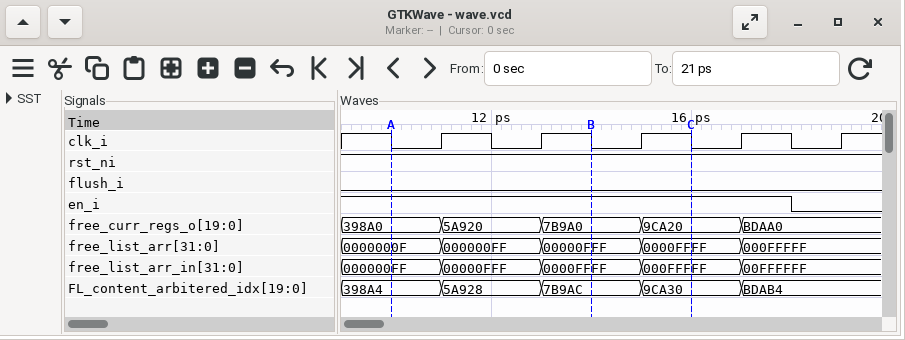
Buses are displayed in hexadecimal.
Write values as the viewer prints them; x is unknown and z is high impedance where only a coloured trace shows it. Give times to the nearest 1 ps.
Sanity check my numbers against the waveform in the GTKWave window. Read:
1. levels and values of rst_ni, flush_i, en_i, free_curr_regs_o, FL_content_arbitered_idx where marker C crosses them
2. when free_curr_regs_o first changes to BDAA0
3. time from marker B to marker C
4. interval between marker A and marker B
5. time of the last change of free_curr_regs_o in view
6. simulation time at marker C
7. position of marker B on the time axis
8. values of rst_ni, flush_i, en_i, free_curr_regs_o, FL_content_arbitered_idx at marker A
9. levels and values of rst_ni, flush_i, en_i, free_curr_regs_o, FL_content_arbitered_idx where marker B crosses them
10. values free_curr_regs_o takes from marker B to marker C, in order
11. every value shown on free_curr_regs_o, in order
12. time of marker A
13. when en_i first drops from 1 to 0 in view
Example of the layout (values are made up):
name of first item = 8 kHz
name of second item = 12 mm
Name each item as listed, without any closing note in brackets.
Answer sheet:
levels and values of rst_ni, flush_i, en_i, free_curr_regs_o, FL_content_arbitered_idx where marker C crosses them = rst_ni=1, flush_i=0, en_i=1, free_curr_regs_o=9CA20, FL_content_arbitered_idx=9CA30
when free_curr_regs_o first changes to BDAA0 = 17 ps
time from marker B to marker C = 2 ps
interval between marker A and marker B = 4 ps
time of the last change of free_curr_regs_o in view = 17 ps
simulation time at marker C = 16 ps
position of marker B on the time axis = 14 ps
values of rst_ni, flush_i, en_i, free_curr_regs_o, FL_content_arbitered_idx at marker A = rst_ni=1, flush_i=0, en_i=1, free_curr_regs_o=398A0, FL_content_arbitered_idx=398A4
levels and values of rst_ni, flush_i, en_i, free_curr_regs_o, FL_content_arbitered_idx where marker B crosses them = rst_ni=1, flush_i=0, en_i=1, free_curr_regs_o=7B9A0, FL_content_arbitered_idx=7B9AC
values free_curr_regs_o takes from marker B to marker C, in order = 7B9A0, 9CA20
every value shown on free_curr_regs_o, in order = 398A0, 5A920, 7B9A0, 9CA20, BDAA0
time of marker A = 10 ps
when en_i first drops from 1 to 0 in view = 18 ps
